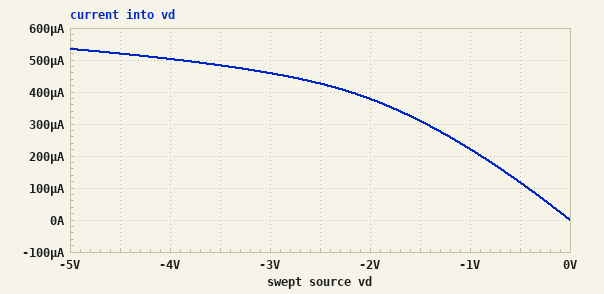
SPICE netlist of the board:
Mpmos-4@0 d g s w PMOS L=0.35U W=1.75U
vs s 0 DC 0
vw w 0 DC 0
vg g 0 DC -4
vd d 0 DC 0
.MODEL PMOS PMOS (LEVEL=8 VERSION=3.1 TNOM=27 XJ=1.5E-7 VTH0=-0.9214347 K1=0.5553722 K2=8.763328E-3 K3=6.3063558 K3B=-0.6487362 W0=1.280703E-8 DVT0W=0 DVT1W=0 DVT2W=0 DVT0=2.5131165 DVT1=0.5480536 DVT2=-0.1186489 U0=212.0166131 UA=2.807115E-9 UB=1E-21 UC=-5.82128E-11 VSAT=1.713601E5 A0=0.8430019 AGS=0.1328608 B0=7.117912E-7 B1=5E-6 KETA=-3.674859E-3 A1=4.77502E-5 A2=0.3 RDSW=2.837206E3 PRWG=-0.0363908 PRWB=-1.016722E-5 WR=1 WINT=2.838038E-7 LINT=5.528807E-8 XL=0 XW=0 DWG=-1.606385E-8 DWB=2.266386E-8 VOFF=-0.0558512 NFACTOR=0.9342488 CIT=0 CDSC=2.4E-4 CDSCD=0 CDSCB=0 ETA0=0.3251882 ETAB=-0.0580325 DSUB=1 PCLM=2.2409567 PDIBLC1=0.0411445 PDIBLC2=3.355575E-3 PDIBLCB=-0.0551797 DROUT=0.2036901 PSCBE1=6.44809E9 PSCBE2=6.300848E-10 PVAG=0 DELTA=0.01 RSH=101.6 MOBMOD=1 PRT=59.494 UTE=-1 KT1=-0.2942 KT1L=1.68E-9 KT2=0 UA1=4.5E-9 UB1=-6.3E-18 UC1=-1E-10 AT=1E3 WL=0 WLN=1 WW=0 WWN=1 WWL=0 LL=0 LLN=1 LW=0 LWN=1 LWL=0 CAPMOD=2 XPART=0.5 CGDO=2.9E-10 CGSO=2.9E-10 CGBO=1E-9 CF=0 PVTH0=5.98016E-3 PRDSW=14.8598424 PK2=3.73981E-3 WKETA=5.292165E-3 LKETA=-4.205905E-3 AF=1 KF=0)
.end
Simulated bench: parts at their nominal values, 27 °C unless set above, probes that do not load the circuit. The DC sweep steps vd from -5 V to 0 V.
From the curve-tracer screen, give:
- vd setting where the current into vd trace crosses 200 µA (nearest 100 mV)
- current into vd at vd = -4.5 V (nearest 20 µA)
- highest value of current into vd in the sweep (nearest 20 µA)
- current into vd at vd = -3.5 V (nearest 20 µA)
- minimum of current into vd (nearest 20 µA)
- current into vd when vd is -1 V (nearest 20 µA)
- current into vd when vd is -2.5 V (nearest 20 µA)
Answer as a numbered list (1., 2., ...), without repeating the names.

1. -900 mV
2. 520 µA
3. 540 µA
4. 480 µA
5. 0 A
6. 220 µA
7. 420 µA
